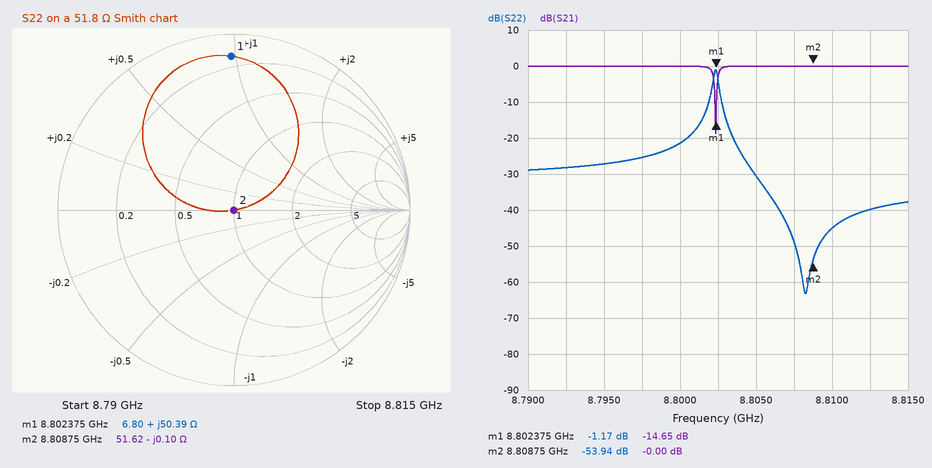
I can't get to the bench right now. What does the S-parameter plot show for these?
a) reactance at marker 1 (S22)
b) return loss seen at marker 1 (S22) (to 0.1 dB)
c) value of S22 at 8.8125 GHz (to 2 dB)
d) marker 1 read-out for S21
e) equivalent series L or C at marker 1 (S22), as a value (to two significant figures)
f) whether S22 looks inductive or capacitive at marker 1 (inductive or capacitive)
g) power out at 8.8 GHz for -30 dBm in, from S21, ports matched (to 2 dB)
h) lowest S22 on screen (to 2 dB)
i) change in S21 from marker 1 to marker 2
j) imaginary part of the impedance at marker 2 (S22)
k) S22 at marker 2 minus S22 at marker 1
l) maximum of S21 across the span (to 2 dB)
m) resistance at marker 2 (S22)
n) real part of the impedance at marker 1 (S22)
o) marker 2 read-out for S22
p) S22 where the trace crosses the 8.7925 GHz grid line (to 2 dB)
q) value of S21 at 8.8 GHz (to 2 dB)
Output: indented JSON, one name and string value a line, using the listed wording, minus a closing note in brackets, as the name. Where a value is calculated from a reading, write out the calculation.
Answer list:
{
  "reactance at marker 1": "+50.39 Ω",
  "return loss seen at marker 1 (S22)": "1.2 dB",
  "value of S22 at 8.8125 GHz": "-40 dB",
  "marker 1 read-out for S21": "-14.65 dB",
  "equivalent series L or C at marker 1 (S22), as a value": "L = 50.39 Ω/(2π × 8.802375 GHz) ≈ 911 pH, so 910 pH to two significant figures",
  "whether S22 looks inductive or capacitive at marker 1": "inductive",
  "power out at 8.8 GHz for -30 dBm in, from S21, ports matched": "-30 dBm + (0 dB) = -30 dBm",
  "lowest S22 on screen": "-64 dB",
  "change in S21 from marker 1 to marker 2": "-0 − (-14.65) = 14.65 dB",
  "imaginary part of the impedance at marker 2": "-0.10 Ω",
  "S22 at marker 2 minus S22 at marker 1": "-53.94 − (-1.17) = -52.77 dB",
  "maximum of S21 across the span": "0 dB",
  "resistance at marker 2": "51.62 Ω",
  "real part of the impedance at marker 1": "6.80 Ω",
  "marker 2 read-out for S22": "-53.94 dB",
  "S22 where the trace crosses the 8.7925 GHz grid line": "-28 dB",
  "value of S21 at 8.8 GHz": "0 dB"
}
